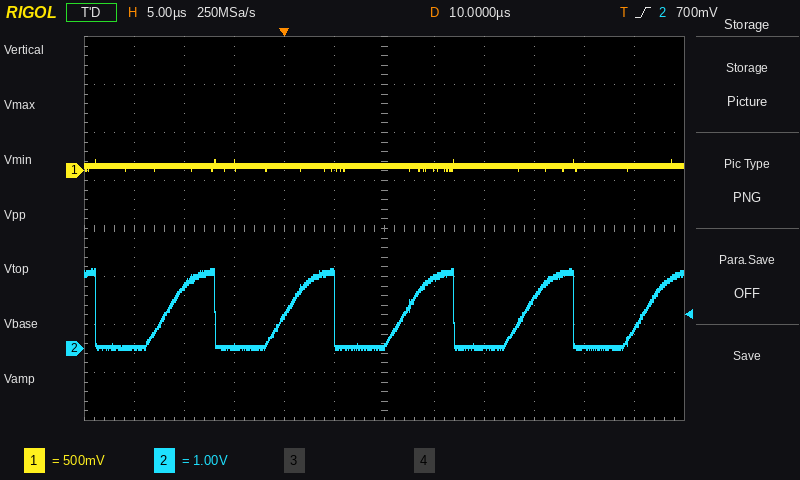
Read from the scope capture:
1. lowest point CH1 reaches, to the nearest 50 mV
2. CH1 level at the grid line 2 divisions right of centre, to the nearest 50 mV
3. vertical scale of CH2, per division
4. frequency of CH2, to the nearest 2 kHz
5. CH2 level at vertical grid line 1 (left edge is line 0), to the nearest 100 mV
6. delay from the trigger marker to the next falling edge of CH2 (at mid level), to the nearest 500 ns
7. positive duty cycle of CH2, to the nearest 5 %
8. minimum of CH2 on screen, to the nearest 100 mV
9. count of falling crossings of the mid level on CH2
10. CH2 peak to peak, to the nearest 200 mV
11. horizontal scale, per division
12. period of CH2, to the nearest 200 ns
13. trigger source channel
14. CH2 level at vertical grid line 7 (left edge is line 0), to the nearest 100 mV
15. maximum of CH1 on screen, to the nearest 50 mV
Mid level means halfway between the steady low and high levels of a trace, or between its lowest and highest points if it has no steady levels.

0 mV
50 mV
1 V
84 kHz
0.0 V
5.0 µs
40 %
0.0 V
5
1.6 V
5 µs
12.0 µs
CH2
1.5 V
100 mV
